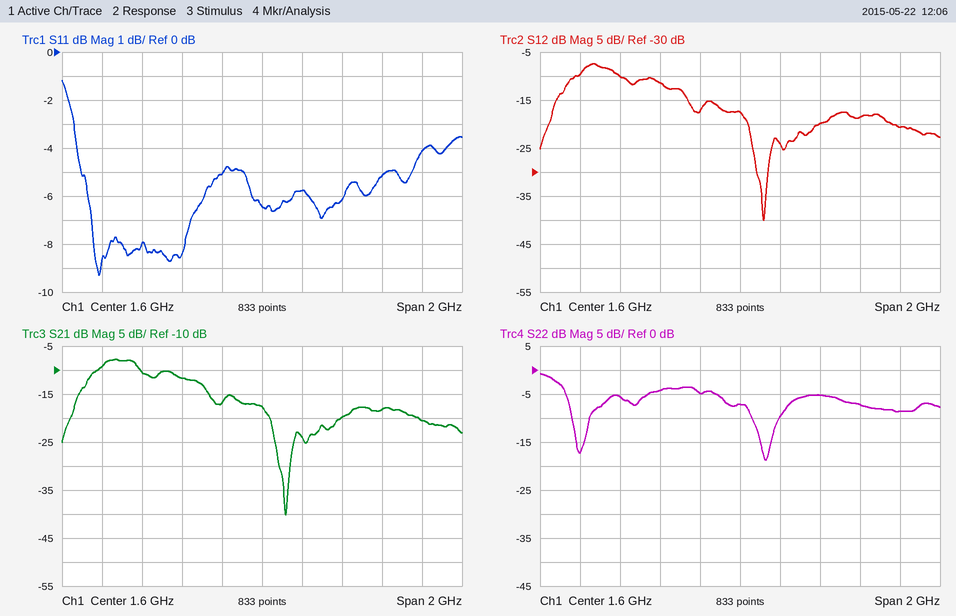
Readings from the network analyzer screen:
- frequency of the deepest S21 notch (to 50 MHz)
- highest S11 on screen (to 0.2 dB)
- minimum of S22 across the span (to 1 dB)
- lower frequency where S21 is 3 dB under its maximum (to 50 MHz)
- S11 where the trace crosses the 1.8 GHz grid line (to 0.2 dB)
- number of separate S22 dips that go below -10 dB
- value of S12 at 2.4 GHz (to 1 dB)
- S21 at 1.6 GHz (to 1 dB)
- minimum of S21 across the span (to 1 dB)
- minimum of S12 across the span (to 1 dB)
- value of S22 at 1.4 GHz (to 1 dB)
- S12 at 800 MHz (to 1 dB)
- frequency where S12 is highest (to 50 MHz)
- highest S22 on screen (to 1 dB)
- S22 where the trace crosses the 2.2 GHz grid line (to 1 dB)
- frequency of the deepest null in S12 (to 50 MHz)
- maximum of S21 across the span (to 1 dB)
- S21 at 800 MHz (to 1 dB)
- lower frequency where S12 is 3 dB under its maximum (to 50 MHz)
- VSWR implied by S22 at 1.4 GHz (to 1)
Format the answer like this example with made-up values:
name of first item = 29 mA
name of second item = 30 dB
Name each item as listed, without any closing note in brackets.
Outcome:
frequency of the deepest S21 notch = 1.70 GHz
highest S11 on screen = -1.2 dB
minimum of S22 across the span = -19 dB
lower frequency where S21 is 3 dB under its maximum = 750 MHz
S11 where the trace crosses the 1.8 GHz grid line = -5.8 dB
number of separate S22 dips that go below -10 dB = 2
value of S12 at 2.4 GHz = -21 dB
S21 at 1.6 GHz = -18 dB
minimum of S21 across the span = -40 dB
minimum of S12 across the span = -40 dB
value of S22 at 1.4 GHz = -5 dB
S12 at 800 MHz = -10 dB
frequency where S12 is highest = 850 MHz
highest S22 on screen = -1 dB
S22 where the trace crosses the 2.2 GHz grid line = -7 dB
frequency of the deepest null in S12 = 1.70 GHz
maximum of S21 across the span = -8 dB
S21 at 800 MHz = -9 dB
lower frequency where S12 is 3 dB under its maximum = 750 MHz
VSWR implied by S22 at 1.4 GHz = 4
